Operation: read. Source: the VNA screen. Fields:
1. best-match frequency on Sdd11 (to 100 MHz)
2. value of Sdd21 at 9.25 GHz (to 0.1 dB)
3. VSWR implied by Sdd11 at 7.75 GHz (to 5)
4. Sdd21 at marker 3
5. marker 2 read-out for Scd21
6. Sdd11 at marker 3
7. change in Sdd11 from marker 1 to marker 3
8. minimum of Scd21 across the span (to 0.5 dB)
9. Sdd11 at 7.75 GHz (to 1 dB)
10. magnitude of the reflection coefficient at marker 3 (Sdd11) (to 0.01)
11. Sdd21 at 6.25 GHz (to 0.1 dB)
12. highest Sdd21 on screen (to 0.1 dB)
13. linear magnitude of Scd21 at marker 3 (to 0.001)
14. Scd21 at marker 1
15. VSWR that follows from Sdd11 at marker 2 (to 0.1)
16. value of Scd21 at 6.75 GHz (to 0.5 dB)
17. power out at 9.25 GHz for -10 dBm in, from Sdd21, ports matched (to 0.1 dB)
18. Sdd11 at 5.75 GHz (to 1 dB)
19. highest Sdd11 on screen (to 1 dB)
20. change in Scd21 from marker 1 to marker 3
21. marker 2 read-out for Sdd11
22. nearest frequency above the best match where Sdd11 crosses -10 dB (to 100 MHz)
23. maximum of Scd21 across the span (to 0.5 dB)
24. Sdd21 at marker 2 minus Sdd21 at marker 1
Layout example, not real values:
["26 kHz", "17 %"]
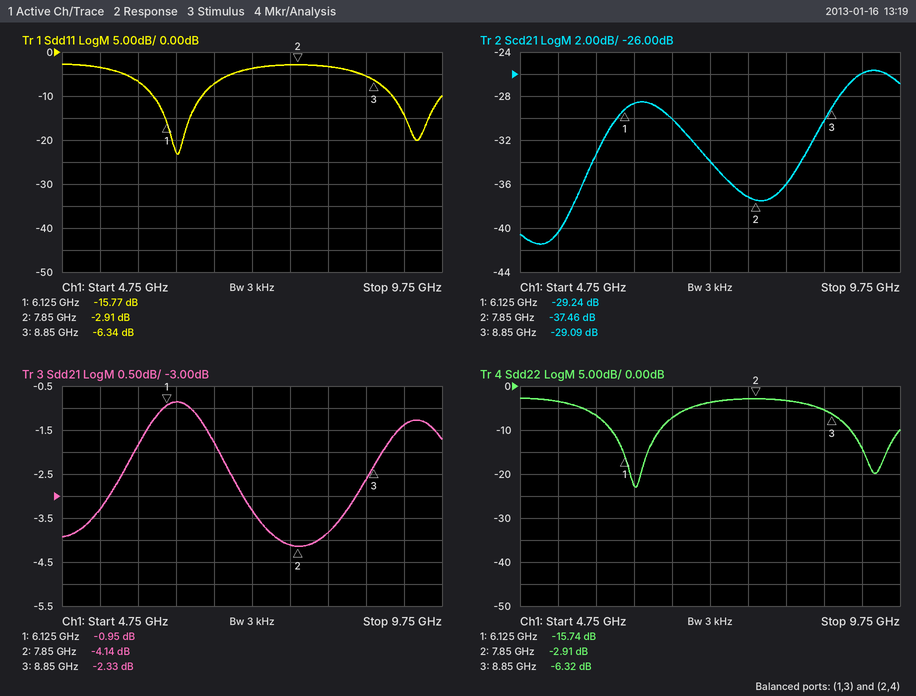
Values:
["6.3 GHz", "-1.4 dB", "5", "-2.33 dB", "-37.46 dB", "-6.34 dB", "9.43 dB", "-41.5 dB", "-3 dB", "0.48", "-0.9 dB", "-0.9 dB", "0.035", "-29.24 dB", "6.0", "-30.0 dB", "-11.4 dBm", "-7 dB", "-3 dB", "0.15 dB", "-2.91 dB", "6.6 GHz", "-25.5 dB", "-3.19 dB"]
